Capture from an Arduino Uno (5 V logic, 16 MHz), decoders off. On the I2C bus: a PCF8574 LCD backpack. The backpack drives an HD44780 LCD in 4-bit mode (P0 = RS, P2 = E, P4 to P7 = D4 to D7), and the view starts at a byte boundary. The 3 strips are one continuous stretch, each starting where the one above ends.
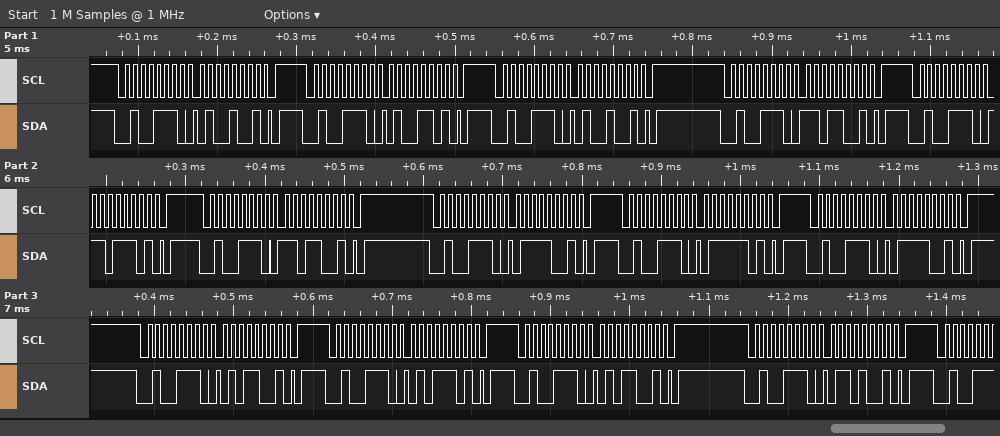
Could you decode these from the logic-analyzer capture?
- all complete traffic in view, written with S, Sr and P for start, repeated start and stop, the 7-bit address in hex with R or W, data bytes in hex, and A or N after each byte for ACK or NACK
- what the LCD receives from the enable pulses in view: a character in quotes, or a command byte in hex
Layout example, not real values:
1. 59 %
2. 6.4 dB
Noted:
1. S 27W A 49 A P S 27W A 4D A P S 27W A 49 A P S 27W A D9 A P S 27W A DD A P S 27W A D9 A P S 27W A 79 A P S 27W A 7D A P S 27W A 79 A P S 27W A 59 A P S 27W A 5D A P S 27W A 59 A P S 27W A 69 A P
2. 'M' 'u'
